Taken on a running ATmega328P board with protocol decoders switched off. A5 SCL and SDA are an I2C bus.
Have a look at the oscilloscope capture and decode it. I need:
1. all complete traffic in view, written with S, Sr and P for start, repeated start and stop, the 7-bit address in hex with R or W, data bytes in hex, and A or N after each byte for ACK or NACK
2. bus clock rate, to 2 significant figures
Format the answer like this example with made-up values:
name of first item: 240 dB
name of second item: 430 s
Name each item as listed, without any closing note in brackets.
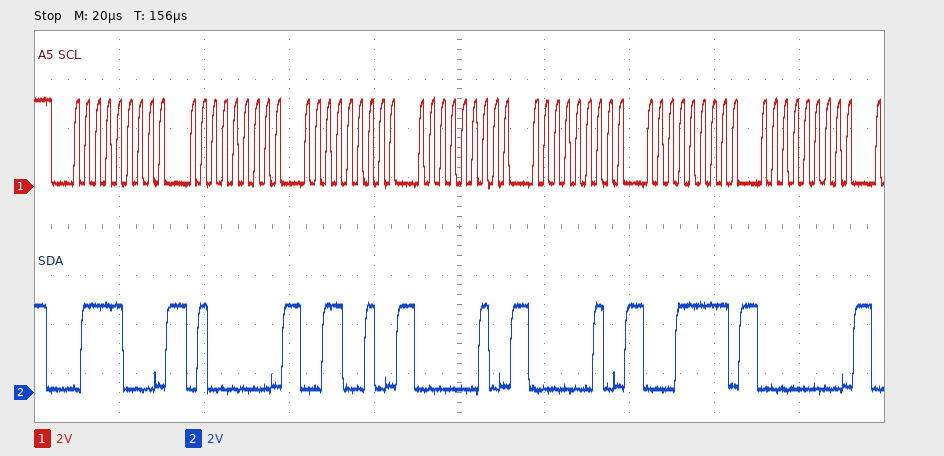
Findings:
all complete traffic in view, written with S, Sr and P for start, repeated start and stop, the 7-bit address in hex with R or W, data bytes in hex, and A or N after each byte for ACK or NACK: S 3CW A 40 A 32 A 02 A 02 A 1F A 00 A
bus clock rate, to 2 significant figures: 400 kHz
